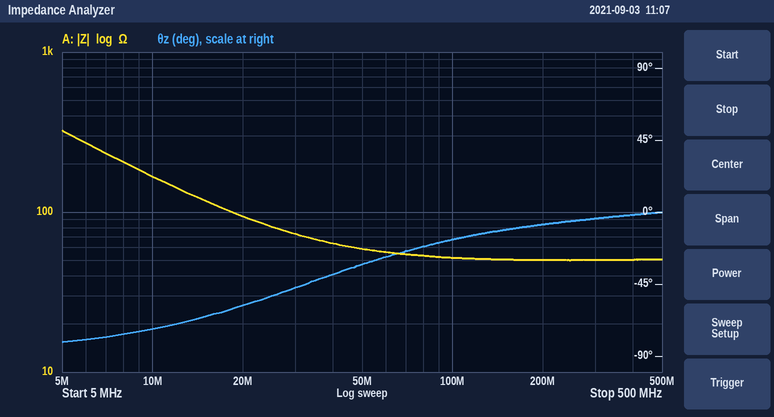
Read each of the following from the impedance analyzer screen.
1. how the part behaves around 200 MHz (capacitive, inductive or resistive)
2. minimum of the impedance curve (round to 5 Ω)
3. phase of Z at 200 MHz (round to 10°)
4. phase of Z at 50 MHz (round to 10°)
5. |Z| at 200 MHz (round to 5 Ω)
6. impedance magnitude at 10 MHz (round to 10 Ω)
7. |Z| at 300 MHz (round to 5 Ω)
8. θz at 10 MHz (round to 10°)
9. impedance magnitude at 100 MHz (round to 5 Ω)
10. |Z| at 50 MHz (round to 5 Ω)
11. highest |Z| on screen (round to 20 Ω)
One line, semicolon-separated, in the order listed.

resistive; 50 Ω; -10°; -30°; 50 Ω; 170 Ω; 50 Ω; -70°; 50 Ω; 60 Ω; 320 Ω
